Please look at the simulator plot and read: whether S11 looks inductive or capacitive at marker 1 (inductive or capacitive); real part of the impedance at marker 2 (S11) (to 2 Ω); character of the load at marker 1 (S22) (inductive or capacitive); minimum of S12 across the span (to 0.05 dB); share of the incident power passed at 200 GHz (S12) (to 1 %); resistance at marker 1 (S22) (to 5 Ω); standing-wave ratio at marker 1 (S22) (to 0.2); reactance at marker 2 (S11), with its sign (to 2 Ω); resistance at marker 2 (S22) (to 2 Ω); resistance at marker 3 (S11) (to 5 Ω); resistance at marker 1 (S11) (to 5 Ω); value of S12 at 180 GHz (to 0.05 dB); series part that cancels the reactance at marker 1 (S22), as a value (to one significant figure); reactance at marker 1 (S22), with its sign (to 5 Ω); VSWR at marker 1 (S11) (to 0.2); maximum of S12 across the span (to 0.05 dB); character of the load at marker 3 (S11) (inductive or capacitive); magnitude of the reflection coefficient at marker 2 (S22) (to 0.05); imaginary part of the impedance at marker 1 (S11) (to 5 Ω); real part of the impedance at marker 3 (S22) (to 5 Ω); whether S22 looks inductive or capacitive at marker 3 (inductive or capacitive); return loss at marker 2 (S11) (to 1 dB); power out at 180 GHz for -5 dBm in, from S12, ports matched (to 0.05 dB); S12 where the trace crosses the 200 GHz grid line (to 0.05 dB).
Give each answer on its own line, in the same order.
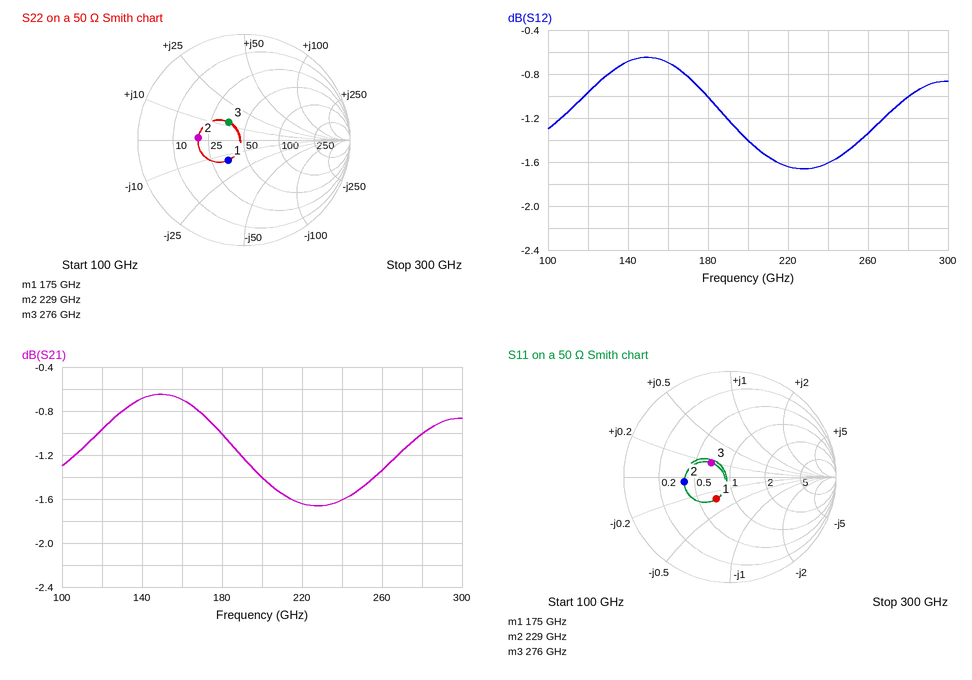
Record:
capacitive
20 Ω
capacitive
-1.65 dB
72 %
35 Ω
1.6
-2 Ω
20 Ω
35 Ω
35 Ω
-1.00 dB
10 pH
-15 Ω
1.6
-0.65 dB
inductive
0.45
-15 Ω
35 Ω
inductive
7 dB
-6.00 dBm
-1.40 dB
